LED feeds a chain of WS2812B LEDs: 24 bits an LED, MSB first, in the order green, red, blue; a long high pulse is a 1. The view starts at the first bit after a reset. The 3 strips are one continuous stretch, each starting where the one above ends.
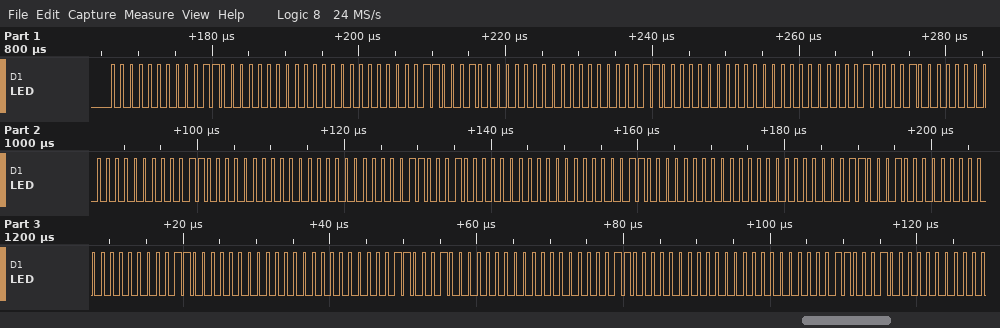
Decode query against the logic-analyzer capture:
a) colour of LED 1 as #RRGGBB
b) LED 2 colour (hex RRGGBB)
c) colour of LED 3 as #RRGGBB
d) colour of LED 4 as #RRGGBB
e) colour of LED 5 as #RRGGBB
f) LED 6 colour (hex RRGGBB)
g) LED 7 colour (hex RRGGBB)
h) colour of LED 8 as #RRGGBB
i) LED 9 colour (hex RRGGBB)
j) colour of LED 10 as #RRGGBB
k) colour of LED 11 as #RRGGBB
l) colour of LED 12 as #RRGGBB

#300000
#310000
#300000
#310000
#300000
#310000
#300000
#310000
#300000
#310000
#300000
#310000
